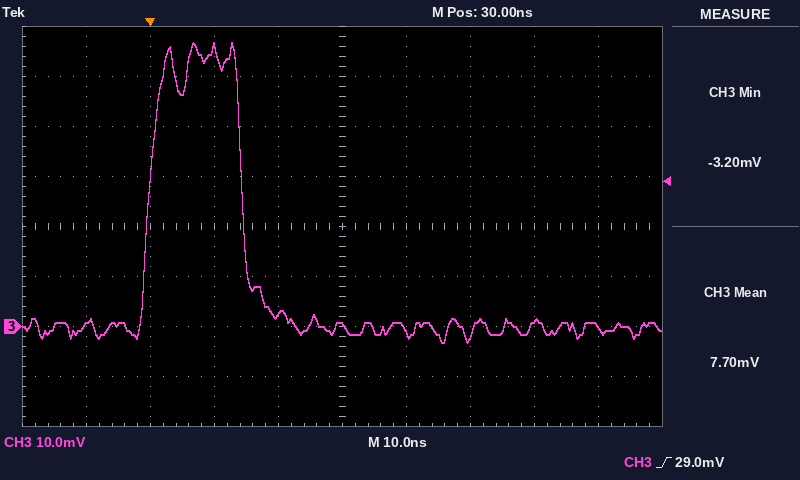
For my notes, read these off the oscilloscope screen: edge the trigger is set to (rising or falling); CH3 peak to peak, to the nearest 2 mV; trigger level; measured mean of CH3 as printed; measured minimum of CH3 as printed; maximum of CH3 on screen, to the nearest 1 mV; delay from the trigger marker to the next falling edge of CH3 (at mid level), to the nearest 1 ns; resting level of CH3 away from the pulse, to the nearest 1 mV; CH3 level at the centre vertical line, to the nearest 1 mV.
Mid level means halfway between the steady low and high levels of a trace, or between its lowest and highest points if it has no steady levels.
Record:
rising
60 mV
29.0 mV
7.70 mV
-3.20 mV
57 mV
14 ns
0 mV
0 mV
